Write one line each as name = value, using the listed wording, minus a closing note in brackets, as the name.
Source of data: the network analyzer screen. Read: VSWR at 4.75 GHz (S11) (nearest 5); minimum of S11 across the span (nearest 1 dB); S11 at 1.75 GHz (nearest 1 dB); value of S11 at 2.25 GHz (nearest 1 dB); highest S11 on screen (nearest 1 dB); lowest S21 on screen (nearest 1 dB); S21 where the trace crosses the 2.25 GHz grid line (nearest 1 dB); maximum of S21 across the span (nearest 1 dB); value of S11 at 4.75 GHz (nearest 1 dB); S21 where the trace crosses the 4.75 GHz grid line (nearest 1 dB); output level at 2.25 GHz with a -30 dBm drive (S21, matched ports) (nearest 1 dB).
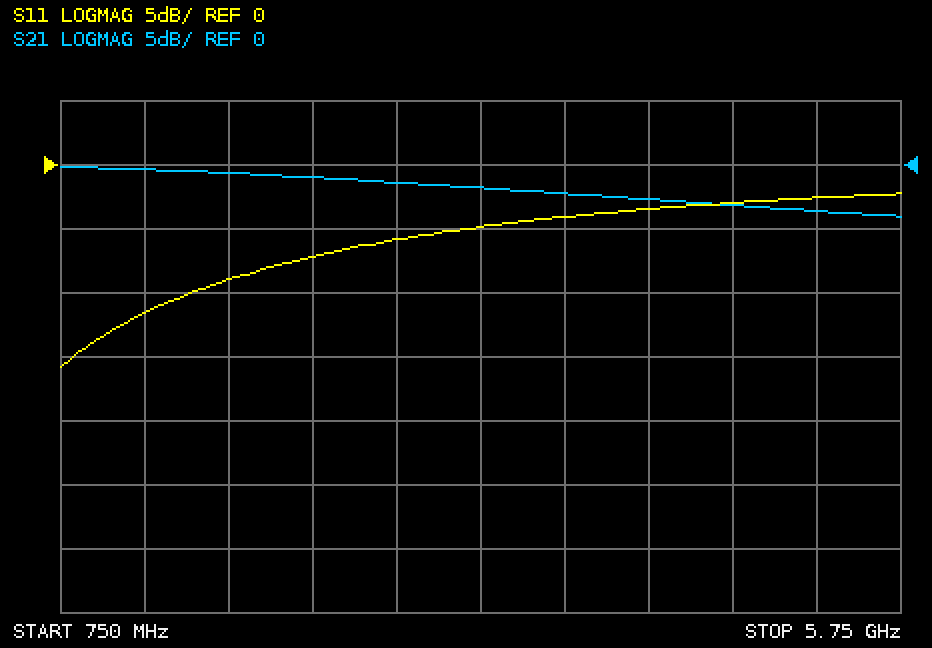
VSWR at 4.75 GHz (S11) = 5
minimum of S11 across the span = -16 dB
S11 at 1.75 GHz = -9 dB
value of S11 at 2.25 GHz = -7 dB
highest S11 on screen = -2 dB
lowest S21 on screen = -4 dB
S21 where the trace crosses the 2.25 GHz grid line = -1 dB
maximum of S21 across the span = 0 dB
value of S11 at 4.75 GHz = -3 dB
S21 where the trace crosses the 4.75 GHz grid line = -3 dB
output level at 2.25 GHz with a -30 dBm drive (S21, matched ports) = -31 dBm
